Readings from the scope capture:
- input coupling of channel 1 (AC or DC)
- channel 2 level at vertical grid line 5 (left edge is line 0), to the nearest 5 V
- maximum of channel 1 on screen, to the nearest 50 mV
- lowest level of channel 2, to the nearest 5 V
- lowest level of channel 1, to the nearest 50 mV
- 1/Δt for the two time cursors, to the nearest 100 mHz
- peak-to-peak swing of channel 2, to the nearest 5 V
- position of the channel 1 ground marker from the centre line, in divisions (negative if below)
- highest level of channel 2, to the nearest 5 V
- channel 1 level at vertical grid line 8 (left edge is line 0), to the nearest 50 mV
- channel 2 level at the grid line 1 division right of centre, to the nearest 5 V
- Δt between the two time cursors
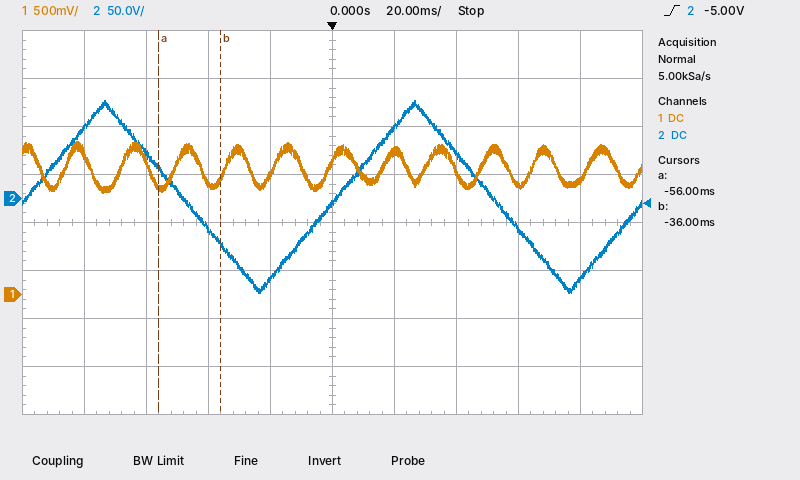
DC
-5 V
1.60 V
-100 V
1.05 V
50.0 Hz
200 V
-1.5 div
100 V
1.15 V
75 V
20 ms
